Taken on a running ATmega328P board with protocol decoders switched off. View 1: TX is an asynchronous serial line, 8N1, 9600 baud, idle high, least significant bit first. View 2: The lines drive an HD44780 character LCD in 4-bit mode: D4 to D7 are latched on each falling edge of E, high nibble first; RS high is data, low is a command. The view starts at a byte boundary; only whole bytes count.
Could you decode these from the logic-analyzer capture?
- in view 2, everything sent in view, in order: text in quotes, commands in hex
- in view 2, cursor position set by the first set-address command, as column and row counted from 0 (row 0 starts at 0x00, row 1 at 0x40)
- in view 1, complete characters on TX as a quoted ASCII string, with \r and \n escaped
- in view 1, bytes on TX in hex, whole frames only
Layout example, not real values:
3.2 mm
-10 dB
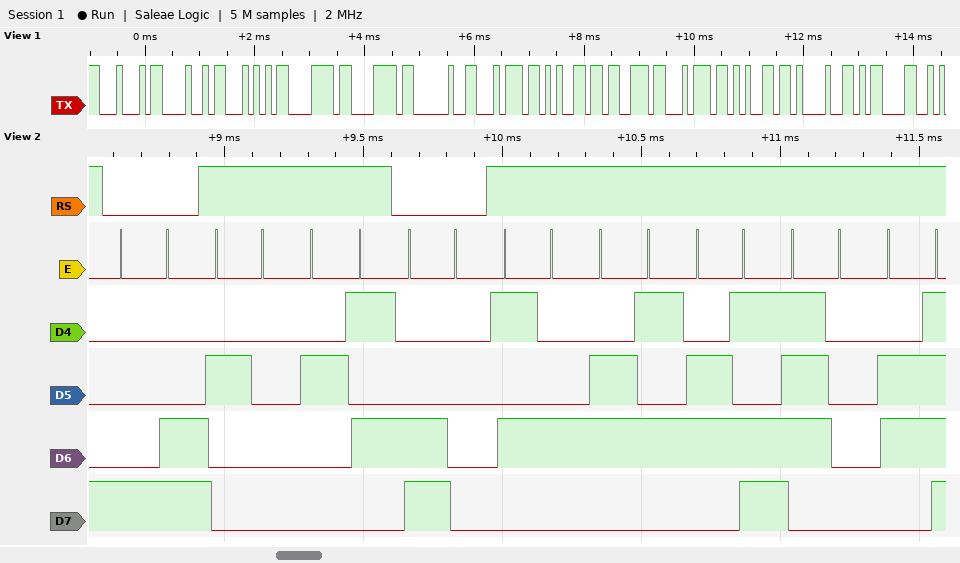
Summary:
0x8C " %" 0xC0 "Tempo"
column 12, row 0
"DHTxx teste!\r"
44 48 54 78 78 20 74 65 73 74 65 21 0D
